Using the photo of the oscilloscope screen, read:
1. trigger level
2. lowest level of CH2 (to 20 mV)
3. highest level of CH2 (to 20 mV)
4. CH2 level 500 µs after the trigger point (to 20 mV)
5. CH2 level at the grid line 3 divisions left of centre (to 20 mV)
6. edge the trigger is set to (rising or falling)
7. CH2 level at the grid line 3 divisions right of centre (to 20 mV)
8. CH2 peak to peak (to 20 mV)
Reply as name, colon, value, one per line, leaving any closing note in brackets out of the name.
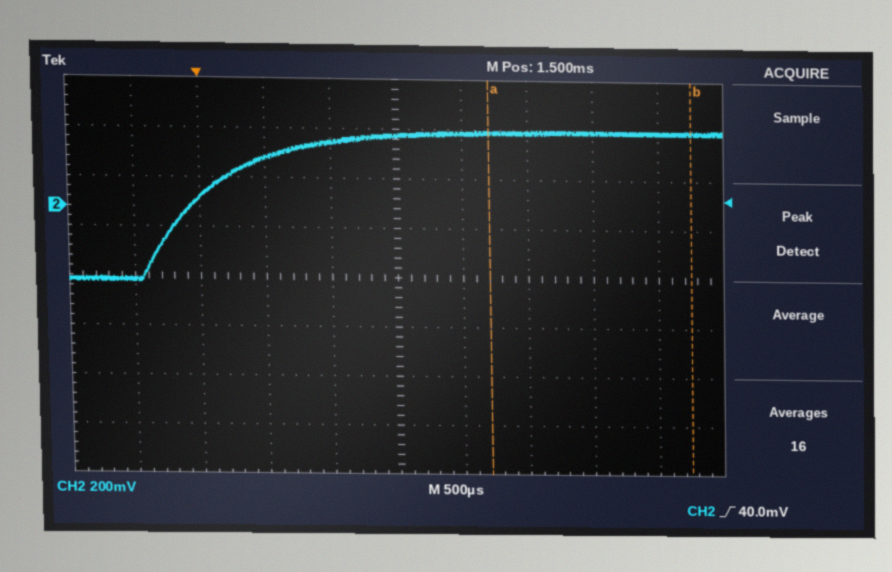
trigger level: 40.0 mV
lowest level of CH2: -300 mV
highest level of CH2: 320 mV
CH2 level 500 µs after the trigger point: 200 mV
CH2 level at the grid line 3 divisions left of centre: 40 mV
edge the trigger is set to: rising
CH2 level at the grid line 3 divisions right of centre: 320 mV
CH2 peak to peak: 620 mV
